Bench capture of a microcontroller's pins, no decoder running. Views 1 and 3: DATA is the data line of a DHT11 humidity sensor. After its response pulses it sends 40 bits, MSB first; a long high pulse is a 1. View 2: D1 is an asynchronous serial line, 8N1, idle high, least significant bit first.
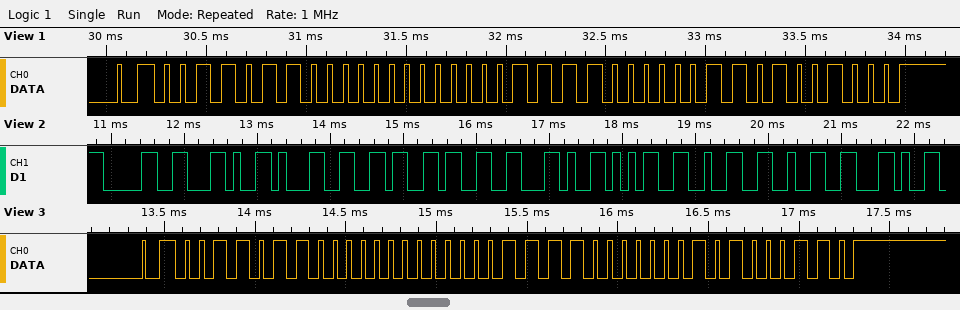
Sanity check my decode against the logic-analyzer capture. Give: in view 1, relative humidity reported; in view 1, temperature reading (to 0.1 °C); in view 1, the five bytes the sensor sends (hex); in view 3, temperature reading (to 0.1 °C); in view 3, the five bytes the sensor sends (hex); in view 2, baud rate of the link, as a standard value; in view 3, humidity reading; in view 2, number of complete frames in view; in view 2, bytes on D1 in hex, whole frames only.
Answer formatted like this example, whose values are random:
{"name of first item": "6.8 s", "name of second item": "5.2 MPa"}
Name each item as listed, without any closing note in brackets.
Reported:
{"in view 1, relative humidity reported": "54 %", "in view 1, temperature reading": "15.3 °C", "in view 1, the five bytes the sensor sends": "36 00 0F 03 48", "in view 3, temperature reading": "15.1 °C", "in view 3, the five bytes the sensor sends": "36 00 0F 01 46", "in view 2, baud rate of the link, as a standard value": "9600 baud", "in view 3, humidity reading": "54 %", "in view 2, number of complete frames in view": "10", "in view 2, bytes on D1 in hex, whole frames only": "30 2C 31 36 33 2C 35 32 32 2C"}
